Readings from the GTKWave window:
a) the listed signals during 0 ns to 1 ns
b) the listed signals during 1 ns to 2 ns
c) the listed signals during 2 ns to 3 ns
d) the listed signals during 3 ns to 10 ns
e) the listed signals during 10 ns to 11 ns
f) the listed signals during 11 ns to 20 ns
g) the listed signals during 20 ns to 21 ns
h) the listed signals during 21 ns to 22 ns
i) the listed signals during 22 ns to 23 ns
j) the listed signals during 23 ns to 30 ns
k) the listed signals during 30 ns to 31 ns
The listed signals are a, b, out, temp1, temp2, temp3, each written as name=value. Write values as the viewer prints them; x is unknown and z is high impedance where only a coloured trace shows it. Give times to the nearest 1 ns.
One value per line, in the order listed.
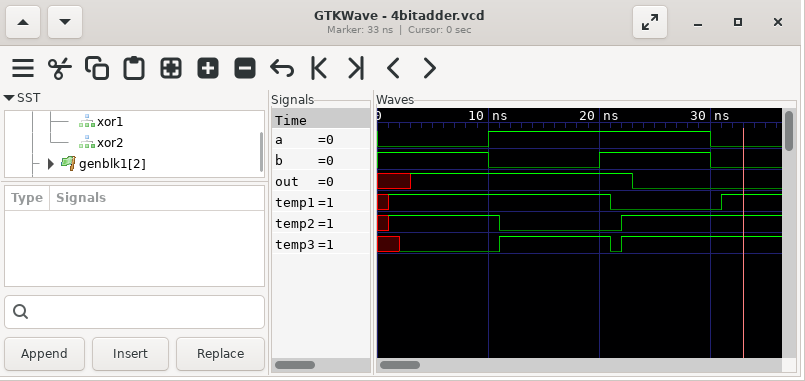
a=0, b=1, out=x, temp1=x, temp2=x, temp3=x
a=0, b=1, out=x, temp1=1, temp2=1, temp3=x
a=0, b=1, out=x, temp1=1, temp2=1, temp3=0
a=0, b=1, out=1, temp1=1, temp2=1, temp3=0
a=1, b=0, out=1, temp1=1, temp2=1, temp3=0
a=1, b=0, out=1, temp1=1, temp2=0, temp3=1
a=1, b=1, out=1, temp1=1, temp2=0, temp3=1
a=1, b=1, out=1, temp1=0, temp2=0, temp3=0
a=1, b=1, out=1, temp1=0, temp2=1, temp3=1
a=1, b=1, out=0, temp1=0, temp2=1, temp3=1
a=0, b=0, out=0, temp1=0, temp2=1, temp3=1
